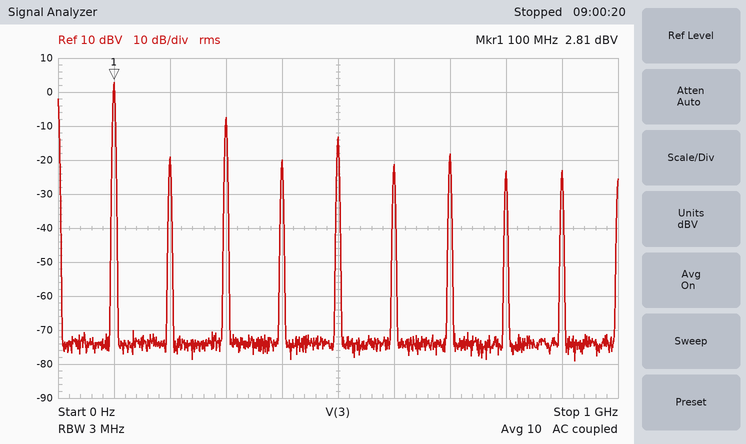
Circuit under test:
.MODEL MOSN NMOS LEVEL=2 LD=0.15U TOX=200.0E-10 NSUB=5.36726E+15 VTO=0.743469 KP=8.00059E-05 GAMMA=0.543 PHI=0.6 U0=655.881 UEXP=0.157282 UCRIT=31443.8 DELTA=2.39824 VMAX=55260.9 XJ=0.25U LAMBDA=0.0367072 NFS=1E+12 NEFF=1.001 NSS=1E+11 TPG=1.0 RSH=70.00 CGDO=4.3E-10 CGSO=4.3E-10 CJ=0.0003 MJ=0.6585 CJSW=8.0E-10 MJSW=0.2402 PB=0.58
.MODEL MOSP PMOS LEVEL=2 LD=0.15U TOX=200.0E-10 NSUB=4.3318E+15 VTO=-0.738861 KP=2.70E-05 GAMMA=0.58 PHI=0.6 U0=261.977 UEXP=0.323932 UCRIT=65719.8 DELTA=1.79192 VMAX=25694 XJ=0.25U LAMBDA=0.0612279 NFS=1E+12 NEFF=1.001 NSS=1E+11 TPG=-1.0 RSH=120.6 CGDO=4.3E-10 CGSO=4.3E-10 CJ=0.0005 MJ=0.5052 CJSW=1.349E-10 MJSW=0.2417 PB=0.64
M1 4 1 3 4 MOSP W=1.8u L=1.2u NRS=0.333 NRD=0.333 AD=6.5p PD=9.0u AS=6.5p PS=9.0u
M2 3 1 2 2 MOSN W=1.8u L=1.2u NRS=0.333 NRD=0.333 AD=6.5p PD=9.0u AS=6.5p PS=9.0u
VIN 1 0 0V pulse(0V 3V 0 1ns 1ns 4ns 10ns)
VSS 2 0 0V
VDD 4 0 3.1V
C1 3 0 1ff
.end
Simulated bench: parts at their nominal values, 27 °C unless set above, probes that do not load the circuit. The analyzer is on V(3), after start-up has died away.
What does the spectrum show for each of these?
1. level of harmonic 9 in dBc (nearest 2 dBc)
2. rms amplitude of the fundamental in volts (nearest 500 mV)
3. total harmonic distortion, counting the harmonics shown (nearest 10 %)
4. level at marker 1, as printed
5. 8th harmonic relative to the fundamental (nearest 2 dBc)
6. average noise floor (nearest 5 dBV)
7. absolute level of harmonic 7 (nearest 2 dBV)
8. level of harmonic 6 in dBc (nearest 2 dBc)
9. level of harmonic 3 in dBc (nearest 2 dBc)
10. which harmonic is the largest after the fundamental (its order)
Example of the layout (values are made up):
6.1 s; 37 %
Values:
-26 dBc; 1.5 V; 40 %; 2.81 dBV; -26 dBc; -75 dBV; -18 dBV; -24 dBc; -10 dBc; 3
